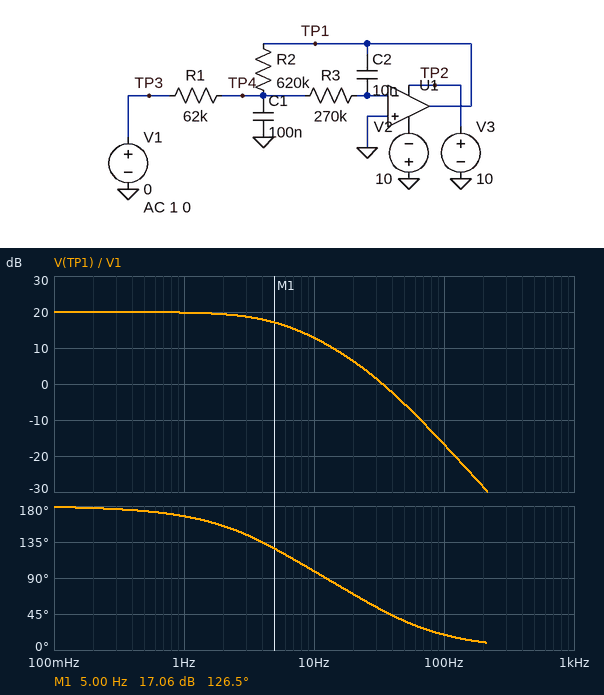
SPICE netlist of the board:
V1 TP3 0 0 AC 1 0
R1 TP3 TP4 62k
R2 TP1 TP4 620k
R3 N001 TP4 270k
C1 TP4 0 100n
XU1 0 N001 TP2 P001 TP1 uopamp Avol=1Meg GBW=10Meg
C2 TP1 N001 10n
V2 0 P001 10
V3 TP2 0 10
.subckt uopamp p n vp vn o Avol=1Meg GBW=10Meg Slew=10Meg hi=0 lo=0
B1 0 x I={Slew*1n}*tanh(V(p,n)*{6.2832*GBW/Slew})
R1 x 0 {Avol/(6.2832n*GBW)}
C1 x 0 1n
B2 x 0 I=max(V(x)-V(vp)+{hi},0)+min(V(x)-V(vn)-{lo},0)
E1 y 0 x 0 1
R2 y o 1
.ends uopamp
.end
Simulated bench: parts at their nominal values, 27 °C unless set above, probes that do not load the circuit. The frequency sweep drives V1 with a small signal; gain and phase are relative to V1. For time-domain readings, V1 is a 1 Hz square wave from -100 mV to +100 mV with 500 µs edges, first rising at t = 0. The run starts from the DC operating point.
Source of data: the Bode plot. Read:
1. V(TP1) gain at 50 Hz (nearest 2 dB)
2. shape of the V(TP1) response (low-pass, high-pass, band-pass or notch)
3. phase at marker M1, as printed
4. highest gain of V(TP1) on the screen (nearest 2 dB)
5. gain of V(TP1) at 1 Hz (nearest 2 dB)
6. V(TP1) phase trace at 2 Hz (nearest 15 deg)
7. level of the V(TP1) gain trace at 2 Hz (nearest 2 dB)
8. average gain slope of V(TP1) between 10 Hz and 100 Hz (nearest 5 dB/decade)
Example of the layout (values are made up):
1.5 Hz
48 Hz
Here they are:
-6 dB
low-pass
126.5 deg
20 dB
20 dB
150 deg
20 dB
-30 dB/decade
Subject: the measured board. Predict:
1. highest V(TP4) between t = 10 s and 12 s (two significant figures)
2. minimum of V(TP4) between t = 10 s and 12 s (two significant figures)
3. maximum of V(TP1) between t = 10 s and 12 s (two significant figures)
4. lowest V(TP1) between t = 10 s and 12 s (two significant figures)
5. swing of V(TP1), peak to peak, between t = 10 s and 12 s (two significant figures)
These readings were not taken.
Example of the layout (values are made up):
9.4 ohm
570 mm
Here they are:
120 mV
-120 mV
1.0 V
-1.0 V
2.0 V
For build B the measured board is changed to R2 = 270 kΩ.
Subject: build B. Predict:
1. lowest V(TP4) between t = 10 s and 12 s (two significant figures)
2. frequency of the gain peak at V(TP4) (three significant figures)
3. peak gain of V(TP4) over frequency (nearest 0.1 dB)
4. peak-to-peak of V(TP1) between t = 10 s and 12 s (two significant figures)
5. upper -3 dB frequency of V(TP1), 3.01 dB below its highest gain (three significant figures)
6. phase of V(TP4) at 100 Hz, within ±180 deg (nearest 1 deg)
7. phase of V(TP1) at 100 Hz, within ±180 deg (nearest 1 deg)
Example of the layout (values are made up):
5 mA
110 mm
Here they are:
-100 mV
18.6 Hz
-3.3 dB
870 mV
11.9 Hz
-69 deg
21 deg
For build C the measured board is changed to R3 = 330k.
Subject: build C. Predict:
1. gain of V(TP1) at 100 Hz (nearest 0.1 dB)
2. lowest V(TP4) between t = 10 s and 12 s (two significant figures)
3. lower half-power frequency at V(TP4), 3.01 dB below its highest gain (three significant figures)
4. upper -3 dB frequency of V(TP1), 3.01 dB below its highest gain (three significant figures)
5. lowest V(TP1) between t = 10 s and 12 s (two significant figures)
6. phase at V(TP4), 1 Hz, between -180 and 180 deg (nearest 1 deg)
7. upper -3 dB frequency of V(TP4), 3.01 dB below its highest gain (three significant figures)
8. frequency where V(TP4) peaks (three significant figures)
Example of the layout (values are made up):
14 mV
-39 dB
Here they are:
-18.5 dB
-130 mV
3.40 Hz
4.21 Hz
-1.0 V
75 deg
36.5 Hz
11.1 Hz
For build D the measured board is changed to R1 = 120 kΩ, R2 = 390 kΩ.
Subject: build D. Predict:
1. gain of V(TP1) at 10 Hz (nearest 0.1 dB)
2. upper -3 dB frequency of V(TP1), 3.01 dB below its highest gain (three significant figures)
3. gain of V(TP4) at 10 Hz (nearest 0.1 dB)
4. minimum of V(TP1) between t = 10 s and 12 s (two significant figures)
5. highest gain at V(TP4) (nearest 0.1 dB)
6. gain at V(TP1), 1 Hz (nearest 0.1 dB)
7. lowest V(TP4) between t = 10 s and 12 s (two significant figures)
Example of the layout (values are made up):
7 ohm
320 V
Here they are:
9.2 dB
14.6 Hz
-6.2 dB
-340 mV
-4.9 dB
10.2 dB
-76 mV
